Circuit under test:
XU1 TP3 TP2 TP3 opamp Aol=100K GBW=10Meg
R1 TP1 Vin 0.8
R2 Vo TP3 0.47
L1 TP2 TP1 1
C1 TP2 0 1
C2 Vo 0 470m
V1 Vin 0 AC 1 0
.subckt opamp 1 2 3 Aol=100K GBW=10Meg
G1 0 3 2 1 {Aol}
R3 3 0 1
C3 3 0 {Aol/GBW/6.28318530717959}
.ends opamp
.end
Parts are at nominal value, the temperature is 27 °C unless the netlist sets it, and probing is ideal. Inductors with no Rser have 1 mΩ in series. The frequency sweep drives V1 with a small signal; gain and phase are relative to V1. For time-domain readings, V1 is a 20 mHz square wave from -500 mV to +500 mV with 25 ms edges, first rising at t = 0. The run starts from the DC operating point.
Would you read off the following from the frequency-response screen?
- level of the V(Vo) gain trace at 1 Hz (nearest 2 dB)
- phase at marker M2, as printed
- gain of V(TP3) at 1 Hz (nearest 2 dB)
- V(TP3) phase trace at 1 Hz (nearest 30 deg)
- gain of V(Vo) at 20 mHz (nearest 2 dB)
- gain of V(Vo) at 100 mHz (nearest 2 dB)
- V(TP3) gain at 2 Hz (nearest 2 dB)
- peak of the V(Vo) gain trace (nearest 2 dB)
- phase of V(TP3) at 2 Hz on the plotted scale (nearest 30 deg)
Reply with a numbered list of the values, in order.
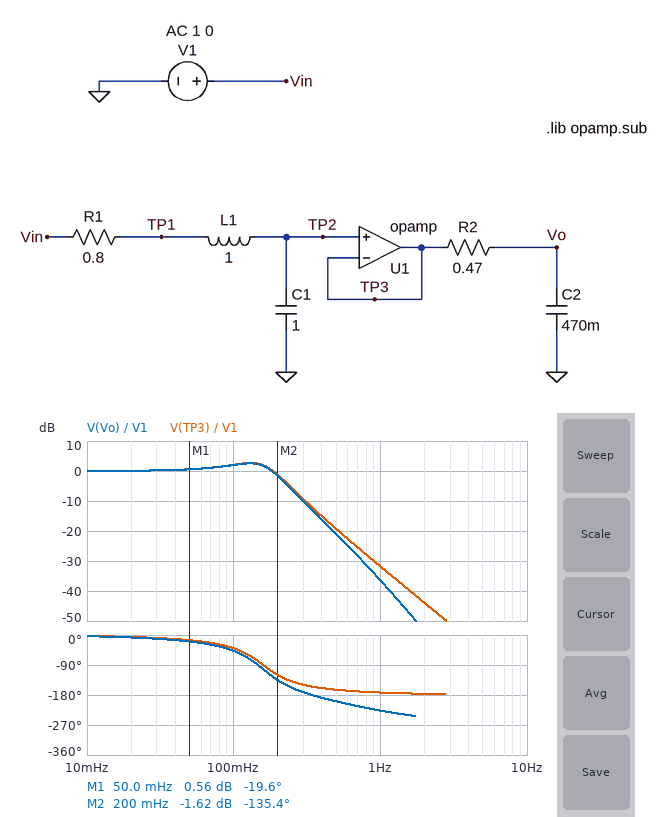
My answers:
1. -36 dB
2. -135.4 deg
3. -32 dB
4. -180 deg
5. 0 dB
6. 2 dB
7. -44 dB
8. 2 dB
9. -180 deg
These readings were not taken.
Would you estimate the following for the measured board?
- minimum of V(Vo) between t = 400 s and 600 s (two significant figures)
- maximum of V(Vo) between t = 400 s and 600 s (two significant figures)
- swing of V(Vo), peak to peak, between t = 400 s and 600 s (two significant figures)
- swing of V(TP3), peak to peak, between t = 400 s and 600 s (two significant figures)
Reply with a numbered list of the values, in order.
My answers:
1. -750 mV
2. 750 mV
3. 1.5 V
4. 1.5 V
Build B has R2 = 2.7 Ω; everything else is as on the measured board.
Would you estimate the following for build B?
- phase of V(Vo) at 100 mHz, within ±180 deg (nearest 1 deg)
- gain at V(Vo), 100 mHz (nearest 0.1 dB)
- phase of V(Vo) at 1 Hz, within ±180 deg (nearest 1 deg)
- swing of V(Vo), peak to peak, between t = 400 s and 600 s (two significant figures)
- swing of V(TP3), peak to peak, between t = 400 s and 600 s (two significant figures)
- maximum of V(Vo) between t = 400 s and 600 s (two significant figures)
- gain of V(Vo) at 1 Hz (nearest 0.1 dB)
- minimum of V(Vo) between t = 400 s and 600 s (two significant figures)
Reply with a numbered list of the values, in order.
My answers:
1. -78 deg
2. -0.1 dB
3. 105 deg
4. 1.2 V
5. 1.5 V
6. 600 mV
7. -49.9 dB
8. -600 mV
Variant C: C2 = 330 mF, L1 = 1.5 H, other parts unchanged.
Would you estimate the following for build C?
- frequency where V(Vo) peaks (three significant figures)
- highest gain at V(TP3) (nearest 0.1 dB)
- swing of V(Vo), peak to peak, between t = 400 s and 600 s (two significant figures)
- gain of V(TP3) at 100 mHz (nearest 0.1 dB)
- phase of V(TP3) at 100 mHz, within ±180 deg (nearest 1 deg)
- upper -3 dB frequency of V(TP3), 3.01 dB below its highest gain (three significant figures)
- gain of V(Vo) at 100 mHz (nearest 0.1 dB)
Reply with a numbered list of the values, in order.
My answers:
1. 115 mHz
2. 4.2 dB
3. 1.7 V
4. 3.8 dB
5. -51 deg
6. 154 mHz
7. 3.7 dB
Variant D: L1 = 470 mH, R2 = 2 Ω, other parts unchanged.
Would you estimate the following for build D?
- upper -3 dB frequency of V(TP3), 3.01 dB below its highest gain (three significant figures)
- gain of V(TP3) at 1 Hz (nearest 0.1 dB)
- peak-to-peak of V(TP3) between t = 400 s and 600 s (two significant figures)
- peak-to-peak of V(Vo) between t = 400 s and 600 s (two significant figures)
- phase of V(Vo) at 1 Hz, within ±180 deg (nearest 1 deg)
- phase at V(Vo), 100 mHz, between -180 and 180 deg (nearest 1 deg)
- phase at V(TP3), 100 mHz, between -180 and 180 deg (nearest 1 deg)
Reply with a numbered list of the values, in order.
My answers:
1. 261 mHz
2. -25.2 dB
3. 1.2 V
4. 1.0 V
5. 116 deg
6. -62 deg
7. -32 deg
